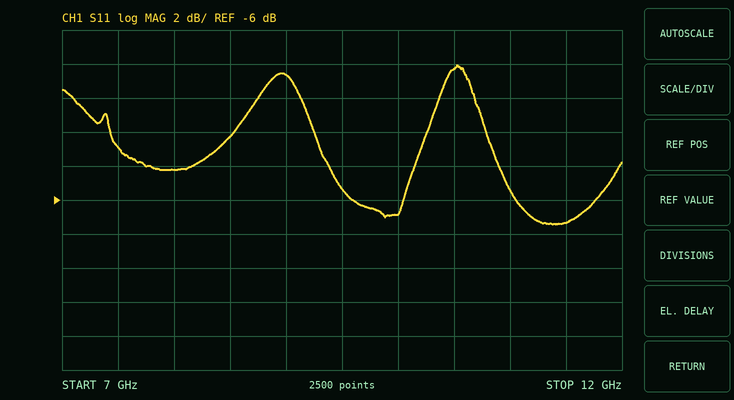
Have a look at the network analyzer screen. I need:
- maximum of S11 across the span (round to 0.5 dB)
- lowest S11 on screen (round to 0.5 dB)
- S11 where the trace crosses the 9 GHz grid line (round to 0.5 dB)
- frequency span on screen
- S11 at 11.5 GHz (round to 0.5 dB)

2.0 dB
-7.5 dB
1.5 dB
5 GHz
-7.5 dB
